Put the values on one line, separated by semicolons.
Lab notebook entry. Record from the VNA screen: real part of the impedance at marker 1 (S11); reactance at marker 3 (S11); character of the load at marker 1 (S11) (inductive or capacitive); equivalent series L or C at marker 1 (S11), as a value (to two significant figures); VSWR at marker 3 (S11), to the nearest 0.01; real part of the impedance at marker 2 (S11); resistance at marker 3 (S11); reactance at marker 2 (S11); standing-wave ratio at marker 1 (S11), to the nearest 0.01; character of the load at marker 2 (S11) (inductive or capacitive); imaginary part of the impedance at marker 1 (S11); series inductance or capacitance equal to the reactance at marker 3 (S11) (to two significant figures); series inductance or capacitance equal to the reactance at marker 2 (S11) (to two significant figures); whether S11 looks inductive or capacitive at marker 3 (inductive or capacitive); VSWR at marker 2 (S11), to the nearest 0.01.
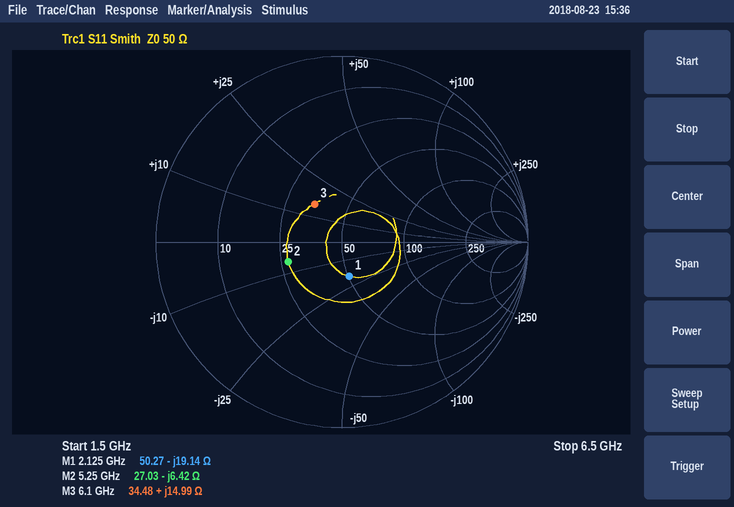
50.27 Ω; +14.99 Ω; capacitive; 3.9 pF; 1.67; 27.03 Ω; 34.48 Ω; -6.42 Ω; 1.46; capacitive; -19.14 Ω; 390 pH; 4.7 pF; inductive; 1.89
